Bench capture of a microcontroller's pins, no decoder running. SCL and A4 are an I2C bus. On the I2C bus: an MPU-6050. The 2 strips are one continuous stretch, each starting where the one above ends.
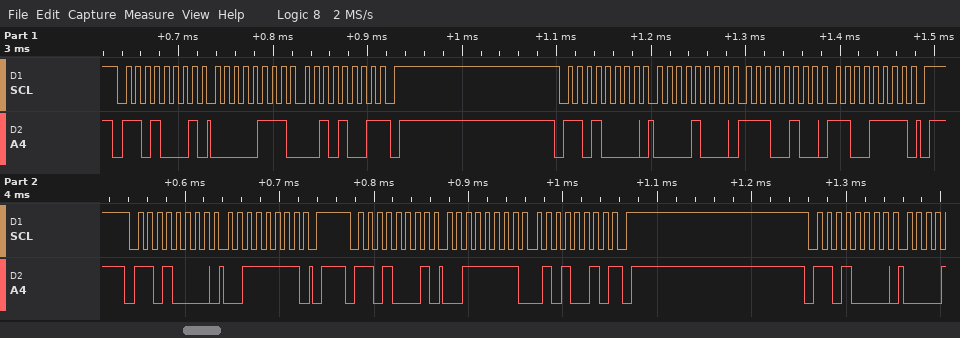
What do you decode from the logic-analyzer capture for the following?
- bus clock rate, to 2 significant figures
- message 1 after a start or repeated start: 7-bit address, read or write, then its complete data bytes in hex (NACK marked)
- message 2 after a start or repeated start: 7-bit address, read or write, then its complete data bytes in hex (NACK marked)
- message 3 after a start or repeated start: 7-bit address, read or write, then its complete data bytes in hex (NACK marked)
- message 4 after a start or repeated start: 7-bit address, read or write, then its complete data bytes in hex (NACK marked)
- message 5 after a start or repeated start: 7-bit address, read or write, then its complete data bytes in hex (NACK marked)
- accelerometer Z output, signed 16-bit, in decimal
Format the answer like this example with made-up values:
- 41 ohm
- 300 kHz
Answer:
- 100 kHz
- 0x68 read: 07 29 NACK
- 0x68 write: 08 E4 CF
- 0x68 write: 3F
- 0x68 read: 3F 52 NACK
- 0x68 write
- 16210
